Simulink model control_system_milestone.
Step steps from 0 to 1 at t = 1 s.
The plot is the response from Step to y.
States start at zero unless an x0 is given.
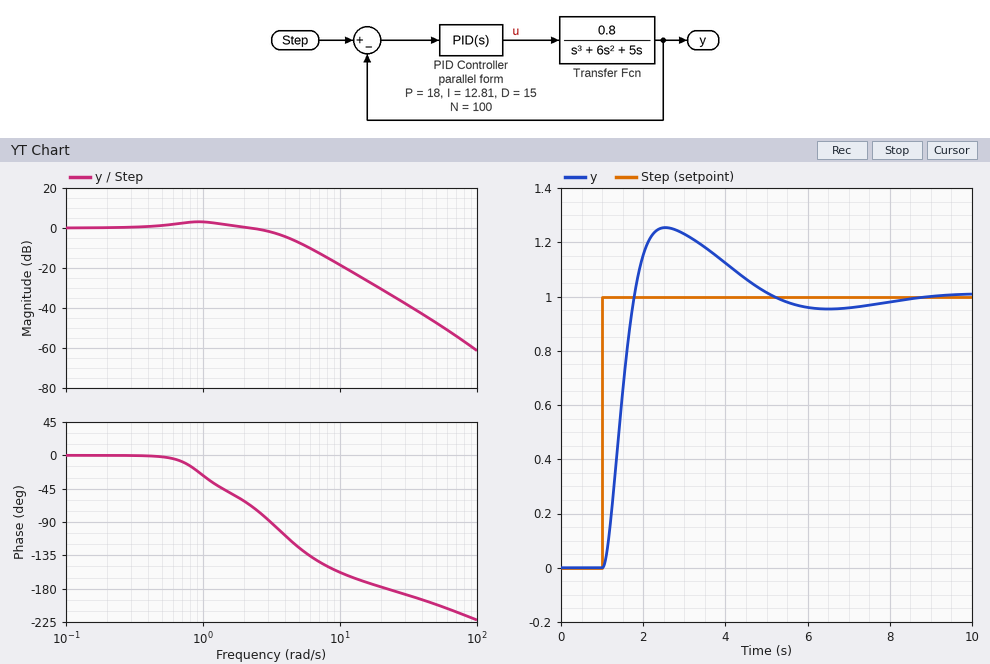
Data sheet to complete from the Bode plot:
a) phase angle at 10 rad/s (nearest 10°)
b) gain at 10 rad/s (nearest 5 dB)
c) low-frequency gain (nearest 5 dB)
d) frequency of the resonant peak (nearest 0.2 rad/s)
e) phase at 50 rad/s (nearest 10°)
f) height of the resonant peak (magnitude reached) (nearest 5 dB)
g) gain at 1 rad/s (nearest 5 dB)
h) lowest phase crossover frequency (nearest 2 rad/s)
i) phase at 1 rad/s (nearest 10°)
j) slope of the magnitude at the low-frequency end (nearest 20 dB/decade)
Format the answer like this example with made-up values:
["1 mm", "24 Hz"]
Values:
["-160°", "-20 dB", "0 dB", "1.0 rad/s", "-200°", "5 dB", "5 dB", "22 rad/s", "-30°", "0 dB/decade"]
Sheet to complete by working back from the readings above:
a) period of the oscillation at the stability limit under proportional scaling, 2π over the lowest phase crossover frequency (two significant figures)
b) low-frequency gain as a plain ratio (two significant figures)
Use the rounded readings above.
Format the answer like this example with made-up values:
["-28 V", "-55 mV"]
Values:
["0.29 s", "1.0"]
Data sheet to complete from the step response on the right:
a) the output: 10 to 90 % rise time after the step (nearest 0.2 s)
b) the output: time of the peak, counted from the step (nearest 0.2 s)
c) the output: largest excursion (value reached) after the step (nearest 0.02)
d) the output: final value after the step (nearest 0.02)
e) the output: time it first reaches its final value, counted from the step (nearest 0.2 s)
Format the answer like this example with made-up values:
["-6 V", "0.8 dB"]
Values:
["0.6 s", "1.6 s", "1.26", "1.00", "0.8 s"]
